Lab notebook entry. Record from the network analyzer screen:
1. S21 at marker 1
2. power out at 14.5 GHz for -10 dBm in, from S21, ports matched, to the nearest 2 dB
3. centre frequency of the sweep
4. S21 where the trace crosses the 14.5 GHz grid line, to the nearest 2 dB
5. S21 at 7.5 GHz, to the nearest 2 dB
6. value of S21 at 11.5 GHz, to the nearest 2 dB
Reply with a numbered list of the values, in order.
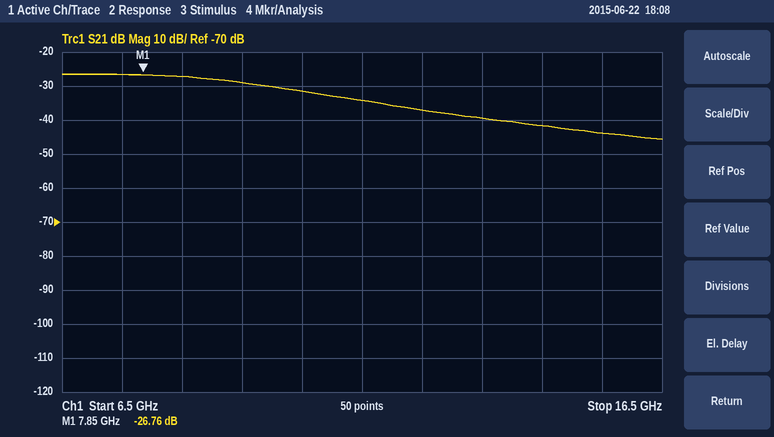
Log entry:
1. -26.76 dB
2. -52 dBm
3. 11.5 GHz
4. -42 dB
5. -26 dB
6. -34 dB
